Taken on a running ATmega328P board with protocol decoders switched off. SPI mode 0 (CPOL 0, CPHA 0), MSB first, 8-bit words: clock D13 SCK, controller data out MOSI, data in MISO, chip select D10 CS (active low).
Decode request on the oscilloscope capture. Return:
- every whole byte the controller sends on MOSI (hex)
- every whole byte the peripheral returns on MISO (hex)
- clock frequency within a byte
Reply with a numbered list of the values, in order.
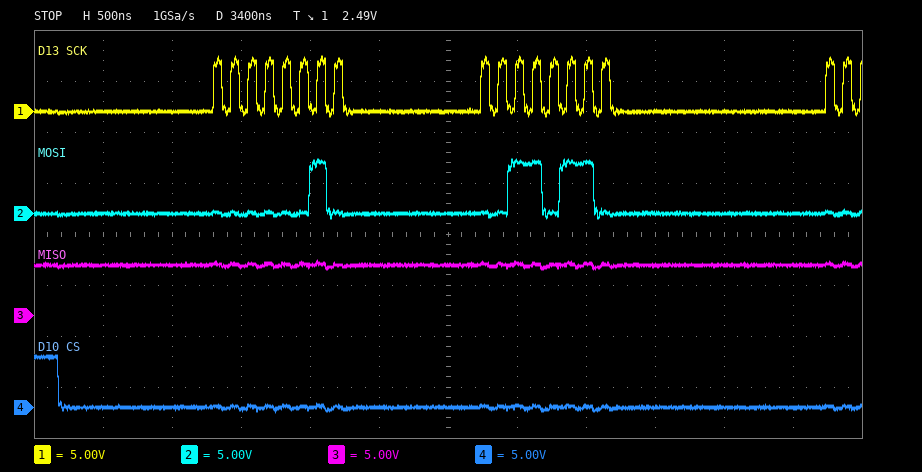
1. 02 36
2. FF FF
3. 8 MHz
